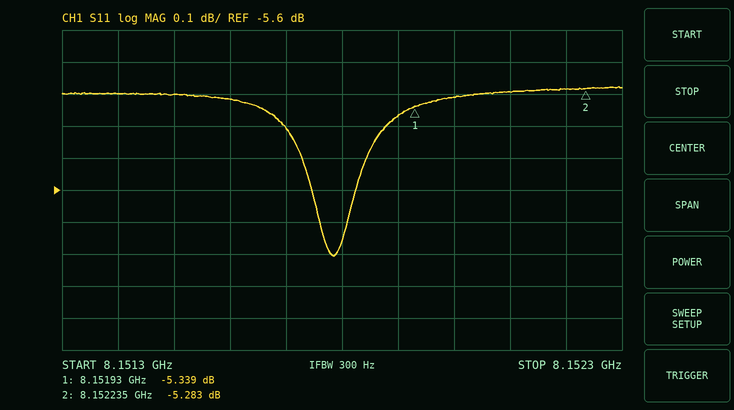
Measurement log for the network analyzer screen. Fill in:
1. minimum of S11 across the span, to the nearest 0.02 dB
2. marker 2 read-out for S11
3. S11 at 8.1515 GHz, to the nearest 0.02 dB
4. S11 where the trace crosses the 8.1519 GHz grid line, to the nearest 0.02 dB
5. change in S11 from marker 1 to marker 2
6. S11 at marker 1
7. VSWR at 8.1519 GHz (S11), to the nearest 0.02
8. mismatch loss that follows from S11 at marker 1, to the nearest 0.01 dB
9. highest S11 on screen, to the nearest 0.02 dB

-5.80 dB
-5.283 dB
-5.30 dB
-5.36 dB
0.056 dB
-5.339 dB
3.34
1.50 dB
-5.28 dB
